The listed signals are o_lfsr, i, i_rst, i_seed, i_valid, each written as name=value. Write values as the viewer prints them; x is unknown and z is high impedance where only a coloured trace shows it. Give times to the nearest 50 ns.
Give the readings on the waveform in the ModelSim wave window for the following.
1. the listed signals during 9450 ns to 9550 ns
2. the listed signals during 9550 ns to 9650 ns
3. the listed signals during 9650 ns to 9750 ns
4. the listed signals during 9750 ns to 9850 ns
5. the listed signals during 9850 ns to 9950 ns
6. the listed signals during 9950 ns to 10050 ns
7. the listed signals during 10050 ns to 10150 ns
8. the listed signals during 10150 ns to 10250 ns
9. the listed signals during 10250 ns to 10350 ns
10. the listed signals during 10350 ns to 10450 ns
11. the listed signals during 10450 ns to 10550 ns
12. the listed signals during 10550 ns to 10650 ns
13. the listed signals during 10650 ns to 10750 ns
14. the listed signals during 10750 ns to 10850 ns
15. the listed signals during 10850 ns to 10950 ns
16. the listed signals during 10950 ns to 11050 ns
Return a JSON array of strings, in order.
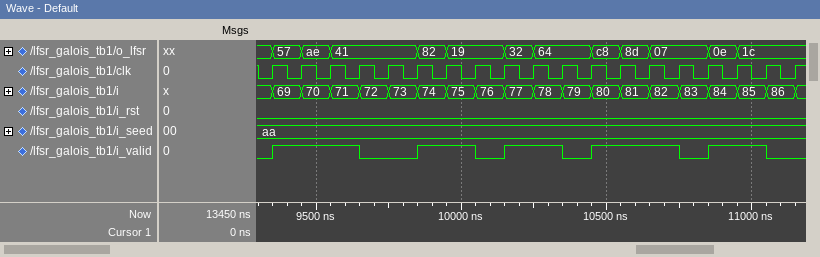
["o_lfsr=ae, i=70, i_rst=0, i_seed=aa, i_valid=1", "o_lfsr=41, i=71, i_rst=0, i_seed=aa, i_valid=1", "o_lfsr=41, i=72, i_rst=0, i_seed=aa, i_valid=0", "o_lfsr=41, i=73, i_rst=0, i_seed=aa, i_valid=0", "o_lfsr=82, i=74, i_rst=0, i_seed=aa, i_valid=1", "o_lfsr=19, i=75, i_rst=0, i_seed=aa, i_valid=1", "o_lfsr=19, i=76, i_rst=0, i_seed=aa, i_valid=0", "o_lfsr=32, i=77, i_rst=0, i_seed=aa, i_valid=1", "o_lfsr=64, i=78, i_rst=0, i_seed=aa, i_valid=1", "o_lfsr=64, i=79, i_rst=0, i_seed=aa, i_valid=0", "o_lfsr=c8, i=80, i_rst=0, i_seed=aa, i_valid=1", "o_lfsr=8d, i=81, i_rst=0, i_seed=aa, i_valid=1", "o_lfsr=07, i=82, i_rst=0, i_seed=aa, i_valid=1", "o_lfsr=07, i=83, i_rst=0, i_seed=aa, i_valid=0", "o_lfsr=0e, i=84, i_rst=0, i_seed=aa, i_valid=1", "o_lfsr=1c, i=85, i_rst=0, i_seed=aa, i_valid=1"]
